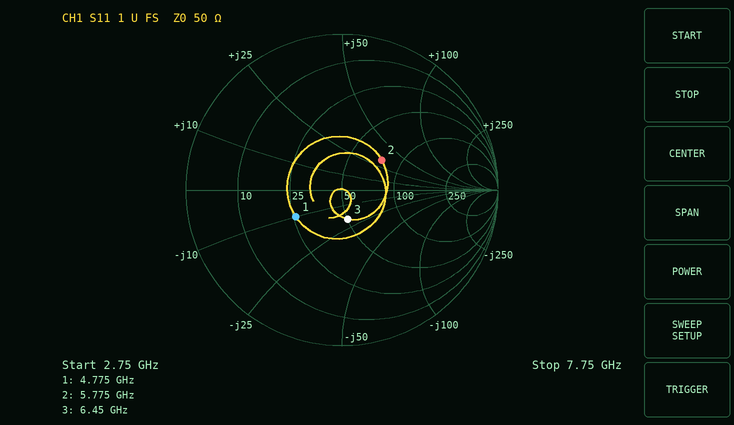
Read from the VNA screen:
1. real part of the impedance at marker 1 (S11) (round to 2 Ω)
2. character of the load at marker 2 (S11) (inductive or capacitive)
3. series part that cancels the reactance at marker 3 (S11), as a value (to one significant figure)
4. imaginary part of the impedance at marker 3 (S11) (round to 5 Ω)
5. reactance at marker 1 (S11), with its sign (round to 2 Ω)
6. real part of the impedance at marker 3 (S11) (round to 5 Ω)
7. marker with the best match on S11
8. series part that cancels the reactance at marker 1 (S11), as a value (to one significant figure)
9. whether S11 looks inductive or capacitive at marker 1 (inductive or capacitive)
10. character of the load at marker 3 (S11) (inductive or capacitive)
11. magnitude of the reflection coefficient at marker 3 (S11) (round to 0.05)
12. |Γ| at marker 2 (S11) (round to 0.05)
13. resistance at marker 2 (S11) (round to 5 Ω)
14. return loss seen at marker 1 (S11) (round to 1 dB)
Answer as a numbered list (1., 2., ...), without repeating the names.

1. 26 Ω
2. inductive
3. 500 pH
4. -20 Ω
5. -10 Ω
6. 50 Ω
7. marker 3
8. 300 pH
9. capacitive
10. capacitive
11. 0.20
12. 0.30
13. 75 Ω
14. 9 dB
